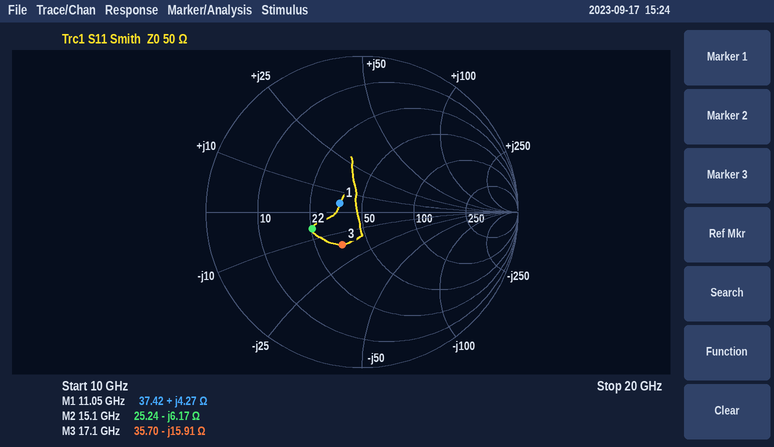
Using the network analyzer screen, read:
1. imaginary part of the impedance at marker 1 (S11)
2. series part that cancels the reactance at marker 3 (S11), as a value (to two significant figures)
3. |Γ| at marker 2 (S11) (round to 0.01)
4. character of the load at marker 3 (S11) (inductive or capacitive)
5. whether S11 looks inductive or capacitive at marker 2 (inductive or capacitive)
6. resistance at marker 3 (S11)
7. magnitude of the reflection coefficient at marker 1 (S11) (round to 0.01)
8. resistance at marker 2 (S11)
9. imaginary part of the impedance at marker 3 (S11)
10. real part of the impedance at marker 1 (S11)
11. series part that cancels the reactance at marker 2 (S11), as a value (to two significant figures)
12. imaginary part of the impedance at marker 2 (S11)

+4.27 Ω
150 pH
0.34
capacitive
capacitive
35.70 Ω
0.15
25.24 Ω
-15.91 Ω
37.42 Ω
65 pH
-6.17 Ω
